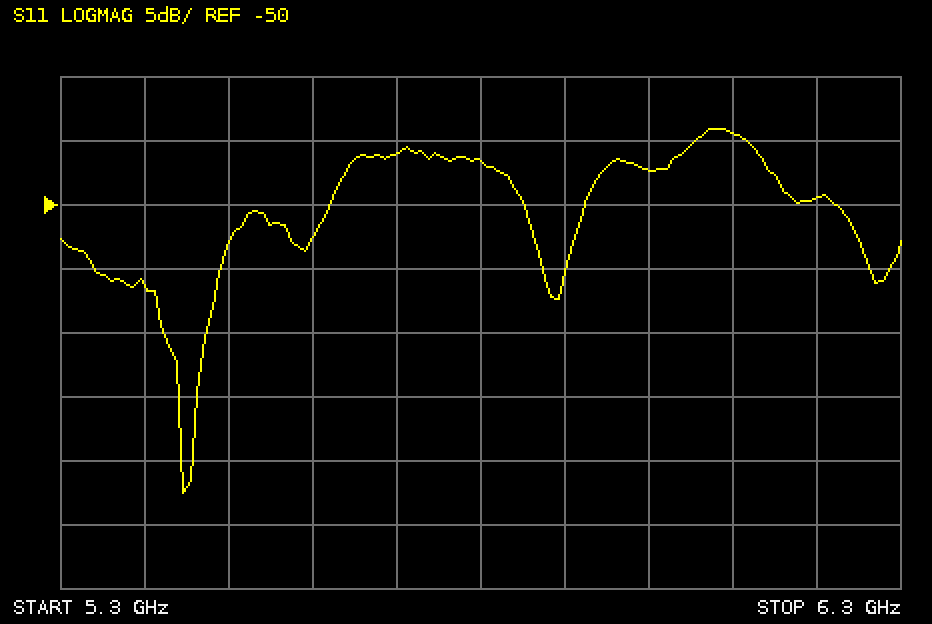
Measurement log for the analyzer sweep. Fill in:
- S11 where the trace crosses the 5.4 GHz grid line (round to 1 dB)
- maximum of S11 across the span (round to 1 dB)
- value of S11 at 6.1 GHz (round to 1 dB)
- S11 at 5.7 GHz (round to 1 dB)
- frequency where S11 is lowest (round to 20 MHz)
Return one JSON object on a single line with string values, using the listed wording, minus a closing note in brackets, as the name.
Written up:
{"S11 where the trace crosses the 5.4 GHz grid line": "-56 dB", "maximum of S11 across the span": "-44 dB", "value of S11 at 6.1 GHz": "-44 dB", "S11 at 5.7 GHz": "-46 dB", "frequency where S11 is lowest": "5.44 GHz"}
